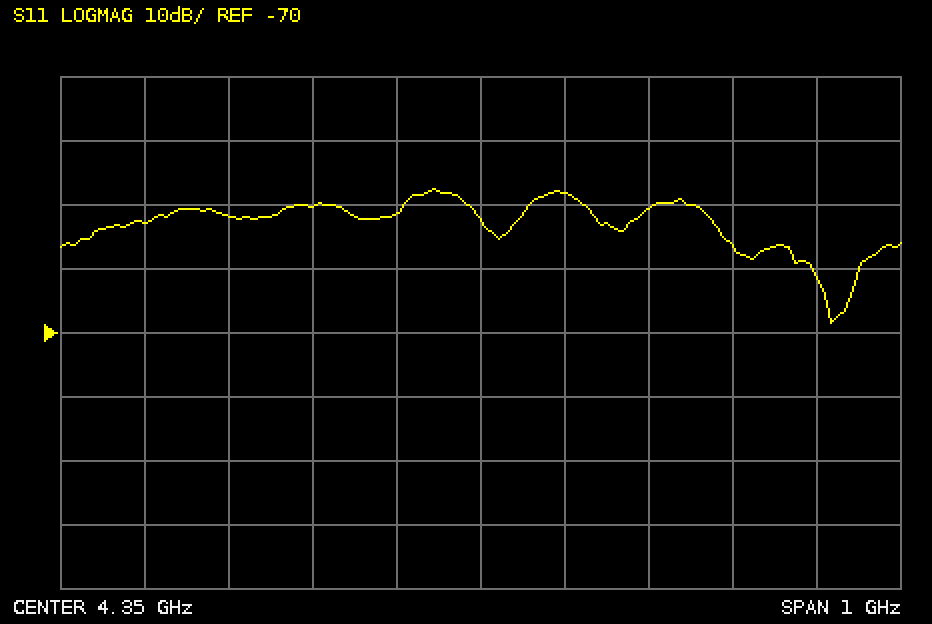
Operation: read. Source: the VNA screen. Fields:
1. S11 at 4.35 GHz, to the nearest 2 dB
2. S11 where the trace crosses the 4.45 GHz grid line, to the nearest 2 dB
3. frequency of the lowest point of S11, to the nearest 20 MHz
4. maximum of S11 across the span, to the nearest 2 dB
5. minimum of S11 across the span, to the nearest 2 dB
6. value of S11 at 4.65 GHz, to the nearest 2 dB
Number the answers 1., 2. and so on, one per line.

1. -52 dB
2. -48 dB
3. 4.76 GHz
4. -48 dB
5. -68 dB
6. -56 dB
